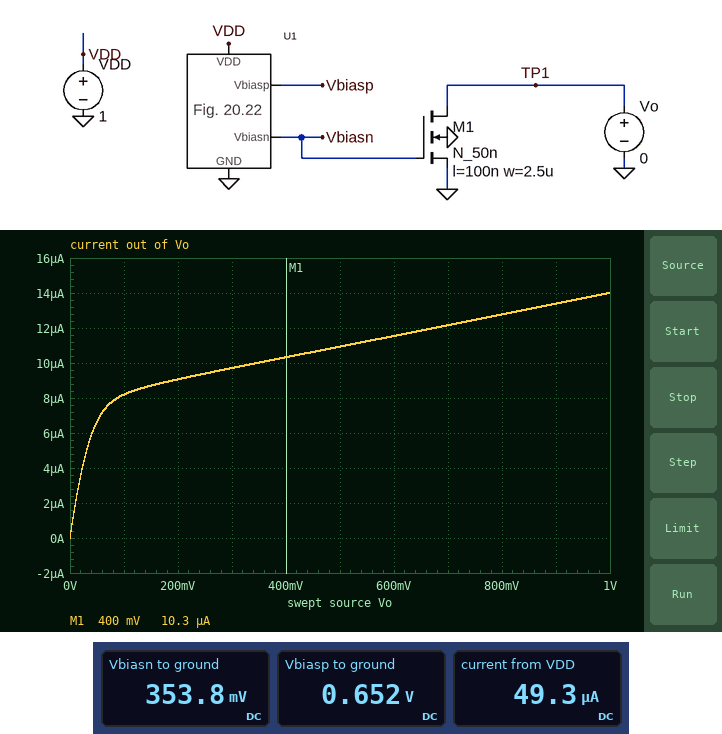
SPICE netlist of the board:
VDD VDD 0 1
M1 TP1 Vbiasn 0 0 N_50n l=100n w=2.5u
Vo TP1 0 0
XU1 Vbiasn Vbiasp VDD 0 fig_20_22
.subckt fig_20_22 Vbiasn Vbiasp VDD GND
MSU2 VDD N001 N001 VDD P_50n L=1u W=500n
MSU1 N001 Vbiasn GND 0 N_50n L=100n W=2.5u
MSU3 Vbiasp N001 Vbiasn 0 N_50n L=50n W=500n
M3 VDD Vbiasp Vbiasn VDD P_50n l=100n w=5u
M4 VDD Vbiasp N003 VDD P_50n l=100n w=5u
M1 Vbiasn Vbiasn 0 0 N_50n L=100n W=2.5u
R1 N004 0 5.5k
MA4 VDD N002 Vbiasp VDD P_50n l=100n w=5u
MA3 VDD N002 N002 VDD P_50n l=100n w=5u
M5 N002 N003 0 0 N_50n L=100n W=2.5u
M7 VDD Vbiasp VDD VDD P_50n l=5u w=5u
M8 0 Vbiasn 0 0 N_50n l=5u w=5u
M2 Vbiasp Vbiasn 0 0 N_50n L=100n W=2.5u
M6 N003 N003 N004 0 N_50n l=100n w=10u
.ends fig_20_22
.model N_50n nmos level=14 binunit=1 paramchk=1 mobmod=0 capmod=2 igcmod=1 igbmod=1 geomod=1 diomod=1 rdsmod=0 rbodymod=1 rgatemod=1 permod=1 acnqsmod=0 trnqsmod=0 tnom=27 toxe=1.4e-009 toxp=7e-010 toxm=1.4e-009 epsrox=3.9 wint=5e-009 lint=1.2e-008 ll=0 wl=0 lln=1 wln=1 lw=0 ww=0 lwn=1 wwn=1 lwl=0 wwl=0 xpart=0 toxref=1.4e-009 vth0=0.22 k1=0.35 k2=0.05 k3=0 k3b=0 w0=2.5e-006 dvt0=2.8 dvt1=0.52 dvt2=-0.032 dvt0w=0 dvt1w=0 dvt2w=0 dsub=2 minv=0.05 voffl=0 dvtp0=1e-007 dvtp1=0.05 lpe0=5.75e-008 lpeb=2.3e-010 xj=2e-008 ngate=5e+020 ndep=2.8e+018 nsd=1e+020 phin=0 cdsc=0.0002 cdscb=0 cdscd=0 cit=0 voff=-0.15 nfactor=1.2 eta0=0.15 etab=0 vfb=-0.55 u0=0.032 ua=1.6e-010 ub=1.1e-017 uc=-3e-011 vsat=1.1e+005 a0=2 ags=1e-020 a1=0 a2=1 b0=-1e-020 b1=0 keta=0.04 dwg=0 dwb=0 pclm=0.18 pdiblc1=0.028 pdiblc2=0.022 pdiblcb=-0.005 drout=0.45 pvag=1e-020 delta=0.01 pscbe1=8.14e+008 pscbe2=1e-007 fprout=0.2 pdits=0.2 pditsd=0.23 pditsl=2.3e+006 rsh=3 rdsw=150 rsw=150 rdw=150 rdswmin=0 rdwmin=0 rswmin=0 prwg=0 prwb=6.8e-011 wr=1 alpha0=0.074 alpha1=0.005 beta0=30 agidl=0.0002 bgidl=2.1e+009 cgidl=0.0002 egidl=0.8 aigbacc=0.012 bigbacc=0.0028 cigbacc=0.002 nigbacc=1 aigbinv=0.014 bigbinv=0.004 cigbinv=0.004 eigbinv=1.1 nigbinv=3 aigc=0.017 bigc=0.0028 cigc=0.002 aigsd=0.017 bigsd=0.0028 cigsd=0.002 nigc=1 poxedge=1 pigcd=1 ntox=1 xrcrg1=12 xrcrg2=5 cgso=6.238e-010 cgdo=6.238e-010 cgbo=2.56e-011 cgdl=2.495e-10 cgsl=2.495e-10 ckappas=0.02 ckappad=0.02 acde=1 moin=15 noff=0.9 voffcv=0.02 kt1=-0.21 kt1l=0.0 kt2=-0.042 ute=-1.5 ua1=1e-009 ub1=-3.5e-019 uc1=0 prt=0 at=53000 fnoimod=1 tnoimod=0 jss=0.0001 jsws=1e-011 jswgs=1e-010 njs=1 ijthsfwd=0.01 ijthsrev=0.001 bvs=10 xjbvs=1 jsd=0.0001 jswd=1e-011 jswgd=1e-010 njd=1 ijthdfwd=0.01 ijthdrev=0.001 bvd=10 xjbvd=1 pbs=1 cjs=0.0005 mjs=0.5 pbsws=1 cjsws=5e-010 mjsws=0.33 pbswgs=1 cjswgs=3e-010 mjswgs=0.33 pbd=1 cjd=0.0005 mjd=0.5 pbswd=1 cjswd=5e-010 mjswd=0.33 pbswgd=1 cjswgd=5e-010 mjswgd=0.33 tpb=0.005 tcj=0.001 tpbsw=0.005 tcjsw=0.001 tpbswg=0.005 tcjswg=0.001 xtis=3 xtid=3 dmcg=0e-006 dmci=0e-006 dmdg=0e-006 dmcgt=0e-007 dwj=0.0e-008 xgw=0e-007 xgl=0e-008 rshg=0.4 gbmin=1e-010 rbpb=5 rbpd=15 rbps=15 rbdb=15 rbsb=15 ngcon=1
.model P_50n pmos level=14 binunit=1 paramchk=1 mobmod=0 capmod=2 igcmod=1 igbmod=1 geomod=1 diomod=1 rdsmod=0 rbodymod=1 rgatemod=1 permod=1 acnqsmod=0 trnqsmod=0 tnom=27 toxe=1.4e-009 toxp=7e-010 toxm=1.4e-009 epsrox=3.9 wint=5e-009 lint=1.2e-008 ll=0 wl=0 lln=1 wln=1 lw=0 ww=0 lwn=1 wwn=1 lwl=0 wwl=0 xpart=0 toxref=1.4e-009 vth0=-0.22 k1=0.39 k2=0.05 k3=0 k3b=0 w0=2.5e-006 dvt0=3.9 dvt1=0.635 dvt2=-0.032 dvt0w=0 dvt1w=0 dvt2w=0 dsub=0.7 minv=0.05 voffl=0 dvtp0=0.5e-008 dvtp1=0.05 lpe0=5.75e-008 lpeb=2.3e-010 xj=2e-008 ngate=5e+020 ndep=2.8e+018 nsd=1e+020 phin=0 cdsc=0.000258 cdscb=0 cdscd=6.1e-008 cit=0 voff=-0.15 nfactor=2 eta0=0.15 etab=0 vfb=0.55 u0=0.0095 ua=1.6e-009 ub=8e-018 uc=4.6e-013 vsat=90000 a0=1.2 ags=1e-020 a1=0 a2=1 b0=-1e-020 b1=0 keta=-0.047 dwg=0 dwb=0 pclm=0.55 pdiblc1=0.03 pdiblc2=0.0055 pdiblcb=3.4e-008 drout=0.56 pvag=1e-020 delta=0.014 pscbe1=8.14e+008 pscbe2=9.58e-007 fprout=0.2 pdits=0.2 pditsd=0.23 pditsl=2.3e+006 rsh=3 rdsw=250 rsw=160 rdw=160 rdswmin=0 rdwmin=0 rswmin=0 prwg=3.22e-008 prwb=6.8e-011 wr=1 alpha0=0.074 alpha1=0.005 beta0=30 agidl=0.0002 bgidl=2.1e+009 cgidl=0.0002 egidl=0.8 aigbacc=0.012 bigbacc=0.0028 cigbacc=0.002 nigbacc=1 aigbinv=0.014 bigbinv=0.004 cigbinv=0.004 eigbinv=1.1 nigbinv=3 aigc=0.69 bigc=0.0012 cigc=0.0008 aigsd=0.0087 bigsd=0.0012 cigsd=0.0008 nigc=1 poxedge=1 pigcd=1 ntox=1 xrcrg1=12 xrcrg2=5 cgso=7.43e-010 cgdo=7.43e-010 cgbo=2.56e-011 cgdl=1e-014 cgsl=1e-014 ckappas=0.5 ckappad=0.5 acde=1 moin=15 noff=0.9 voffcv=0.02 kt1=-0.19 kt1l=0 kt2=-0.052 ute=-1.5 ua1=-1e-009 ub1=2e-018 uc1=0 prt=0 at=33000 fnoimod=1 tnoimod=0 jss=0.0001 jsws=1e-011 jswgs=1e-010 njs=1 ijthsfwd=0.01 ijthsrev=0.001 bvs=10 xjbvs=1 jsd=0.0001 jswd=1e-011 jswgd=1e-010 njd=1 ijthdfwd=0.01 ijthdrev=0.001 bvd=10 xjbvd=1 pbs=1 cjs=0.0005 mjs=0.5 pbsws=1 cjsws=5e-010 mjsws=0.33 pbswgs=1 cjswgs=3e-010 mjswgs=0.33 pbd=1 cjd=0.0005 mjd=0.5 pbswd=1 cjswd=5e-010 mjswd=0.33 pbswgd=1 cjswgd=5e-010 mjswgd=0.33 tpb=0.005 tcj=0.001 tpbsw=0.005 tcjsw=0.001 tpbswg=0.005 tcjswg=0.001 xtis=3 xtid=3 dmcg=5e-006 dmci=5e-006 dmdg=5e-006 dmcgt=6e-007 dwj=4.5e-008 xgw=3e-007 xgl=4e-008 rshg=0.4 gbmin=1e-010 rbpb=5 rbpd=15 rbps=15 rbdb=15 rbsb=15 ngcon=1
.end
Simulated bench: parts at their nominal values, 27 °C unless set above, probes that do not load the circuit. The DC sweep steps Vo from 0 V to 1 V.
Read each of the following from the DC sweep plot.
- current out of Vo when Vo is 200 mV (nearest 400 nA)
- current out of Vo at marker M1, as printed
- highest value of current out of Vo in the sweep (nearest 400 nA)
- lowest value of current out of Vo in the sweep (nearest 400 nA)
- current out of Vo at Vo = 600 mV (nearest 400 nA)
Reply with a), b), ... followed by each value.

a) 9.2 µA
b) 10.3 µA
c) 14.0 µA
d) 0 A
e) 11.6 µA
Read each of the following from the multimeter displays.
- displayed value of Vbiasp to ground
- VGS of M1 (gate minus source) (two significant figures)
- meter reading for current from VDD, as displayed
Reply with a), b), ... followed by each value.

a) 0.652 V
b) 350 mV
c) 49.3 µA
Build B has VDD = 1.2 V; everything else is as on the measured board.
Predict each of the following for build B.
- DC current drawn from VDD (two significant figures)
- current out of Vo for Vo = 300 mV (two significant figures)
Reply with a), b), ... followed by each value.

a) 54 µA
b) 9.8 µA
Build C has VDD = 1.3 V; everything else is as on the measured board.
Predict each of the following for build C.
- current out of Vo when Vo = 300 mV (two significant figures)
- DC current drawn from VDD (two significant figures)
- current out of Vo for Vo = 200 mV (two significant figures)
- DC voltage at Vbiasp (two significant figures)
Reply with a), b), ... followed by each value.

a) 9.8 µA
b) 56 µA
c) 9.2 µA
d) 960 mV
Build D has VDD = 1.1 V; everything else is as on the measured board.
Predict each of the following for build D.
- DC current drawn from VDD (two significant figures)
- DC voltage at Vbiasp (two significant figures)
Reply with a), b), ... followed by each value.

a) 51 µA
b) 750 mV
